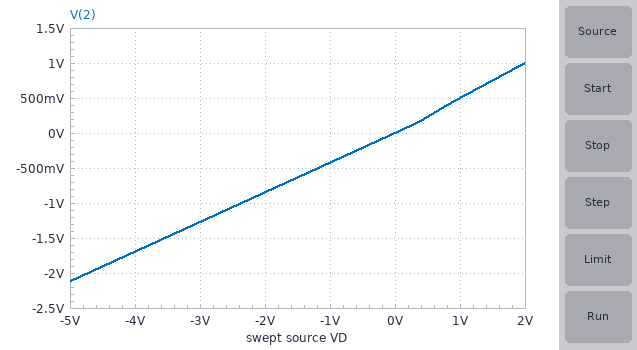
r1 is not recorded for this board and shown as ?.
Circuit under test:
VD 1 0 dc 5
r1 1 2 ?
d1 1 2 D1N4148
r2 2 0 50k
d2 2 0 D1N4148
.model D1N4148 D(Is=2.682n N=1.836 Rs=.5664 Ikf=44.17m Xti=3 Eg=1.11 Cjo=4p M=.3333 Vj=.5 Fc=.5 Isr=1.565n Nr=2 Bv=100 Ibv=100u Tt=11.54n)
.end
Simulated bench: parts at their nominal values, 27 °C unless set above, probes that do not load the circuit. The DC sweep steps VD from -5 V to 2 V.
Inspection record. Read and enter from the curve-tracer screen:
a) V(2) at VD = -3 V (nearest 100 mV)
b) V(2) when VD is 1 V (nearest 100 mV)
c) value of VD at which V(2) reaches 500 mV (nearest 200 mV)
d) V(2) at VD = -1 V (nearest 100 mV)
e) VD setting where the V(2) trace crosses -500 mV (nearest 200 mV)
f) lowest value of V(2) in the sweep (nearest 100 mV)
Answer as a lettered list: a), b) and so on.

a) -1.3 V
b) 500 mV
c) 1.0 V
d) -400 mV
e) -1.2 V
f) -2.1 V
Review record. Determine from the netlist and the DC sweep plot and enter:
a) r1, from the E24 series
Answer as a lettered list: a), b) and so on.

a) 68 kΩ
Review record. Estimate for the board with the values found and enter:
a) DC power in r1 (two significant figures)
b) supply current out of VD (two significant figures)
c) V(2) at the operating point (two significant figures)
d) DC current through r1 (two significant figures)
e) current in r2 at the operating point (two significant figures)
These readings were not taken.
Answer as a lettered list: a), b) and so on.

a) 92 µW
b) 2.4 A
c) 2.5 V
d) 37 µA
e) 50 µA
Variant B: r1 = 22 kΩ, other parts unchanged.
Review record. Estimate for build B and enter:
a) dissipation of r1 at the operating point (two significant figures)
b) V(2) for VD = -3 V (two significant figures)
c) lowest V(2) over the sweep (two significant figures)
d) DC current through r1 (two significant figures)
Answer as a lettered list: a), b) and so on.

a) 280 µW
b) -2.1 V
c) -3.5 V
d) 110 µA
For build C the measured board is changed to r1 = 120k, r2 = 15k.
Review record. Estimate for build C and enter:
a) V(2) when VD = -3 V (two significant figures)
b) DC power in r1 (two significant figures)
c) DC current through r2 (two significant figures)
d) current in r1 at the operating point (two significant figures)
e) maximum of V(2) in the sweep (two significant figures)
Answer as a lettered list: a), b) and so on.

a) -330 mV
b) 52 µW
c) 170 µA
d) 21 µA
e) 1.0 V
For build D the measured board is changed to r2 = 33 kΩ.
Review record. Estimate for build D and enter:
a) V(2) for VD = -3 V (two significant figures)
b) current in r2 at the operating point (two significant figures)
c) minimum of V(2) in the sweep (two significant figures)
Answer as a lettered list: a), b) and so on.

a) -980 mV
b) 76 µA
c) -1.6 V
